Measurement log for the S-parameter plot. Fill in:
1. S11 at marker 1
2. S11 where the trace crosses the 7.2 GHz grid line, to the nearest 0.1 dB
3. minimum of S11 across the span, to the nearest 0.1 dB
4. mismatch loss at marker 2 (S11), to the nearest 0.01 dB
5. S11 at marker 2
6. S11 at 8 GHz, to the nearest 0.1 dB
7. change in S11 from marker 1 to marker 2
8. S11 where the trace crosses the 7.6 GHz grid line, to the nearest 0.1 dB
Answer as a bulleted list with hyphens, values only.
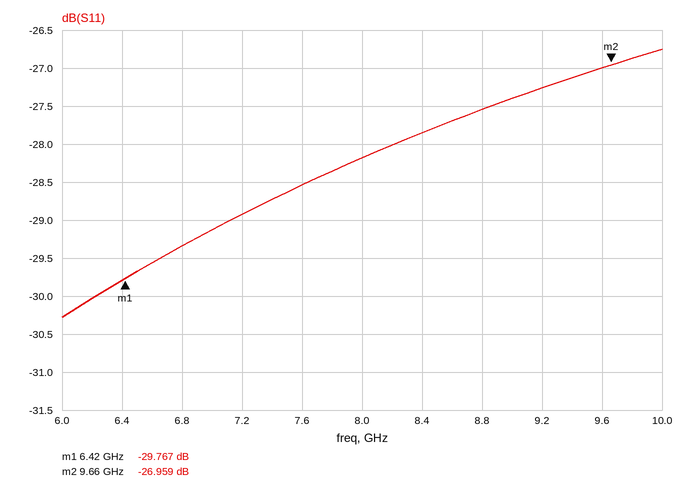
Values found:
- -29.767 dB
- -28.9 dB
- -30.3 dB
- 0.01 dB
- -26.959 dB
- -28.2 dB
- 2.808 dB
- -28.5 dB
